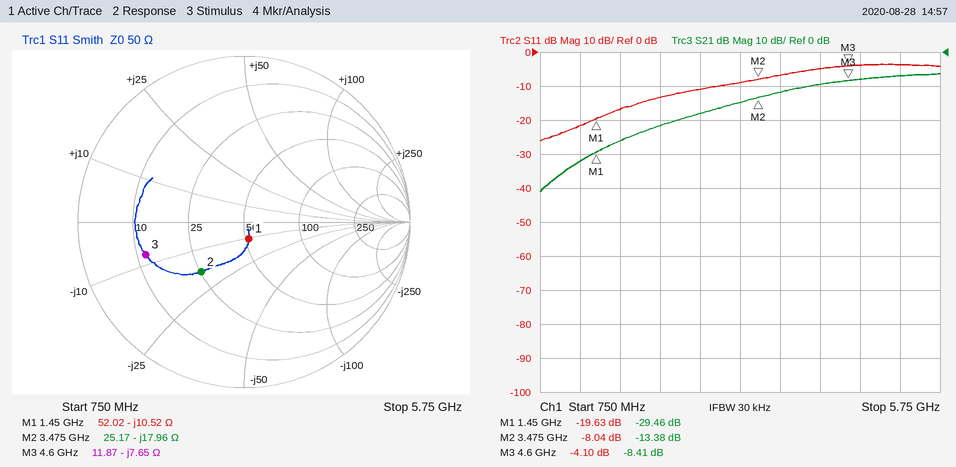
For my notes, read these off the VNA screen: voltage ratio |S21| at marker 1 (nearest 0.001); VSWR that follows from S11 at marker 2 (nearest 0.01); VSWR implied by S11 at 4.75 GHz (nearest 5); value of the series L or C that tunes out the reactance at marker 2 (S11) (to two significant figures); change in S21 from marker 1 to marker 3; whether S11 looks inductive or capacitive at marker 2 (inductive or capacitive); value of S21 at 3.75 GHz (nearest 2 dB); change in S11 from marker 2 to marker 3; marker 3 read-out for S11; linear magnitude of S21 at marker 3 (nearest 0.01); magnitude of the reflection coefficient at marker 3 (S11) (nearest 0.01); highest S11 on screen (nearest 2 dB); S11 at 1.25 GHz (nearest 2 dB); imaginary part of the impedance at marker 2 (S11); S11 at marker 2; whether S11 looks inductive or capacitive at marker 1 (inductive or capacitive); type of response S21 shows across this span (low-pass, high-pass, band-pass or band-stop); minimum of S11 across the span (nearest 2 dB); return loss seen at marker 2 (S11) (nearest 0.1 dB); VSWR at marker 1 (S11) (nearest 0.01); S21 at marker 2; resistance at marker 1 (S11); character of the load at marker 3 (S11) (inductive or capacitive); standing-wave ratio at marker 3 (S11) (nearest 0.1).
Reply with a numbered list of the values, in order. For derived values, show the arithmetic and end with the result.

1. 10^(-29.46/20) ≈ 0.034
2. (1 + 0.3963)/(1 − 0.3963) ≈ 2.31
3. |Γ| = 10^(-4/20) = 0.6310; VSWR = (1 + 0.6310)/(1 − 0.6310) ≈ 4.42, so 5 to the nearest 5
4. L = 17.96 Ω/(2π × 3.475 GHz) ≈ 823 pH, so 820 pH to two significant figures
5. -8.41 − (-29.46) = 21.05 dB
6. capacitive
7. -12 dB
8. -4.1 − (-8.04) = 3.94 dB
9. -4.10 dB
10. 10^(-8.41/20) ≈ 0.38
11. 10^(-4.1/20) ≈ 0.62
12. -4 dB
13. -22 dB
14. -17.96 Ω
15. -8.04 dB
16. capacitive
17. high-pass
18. -26 dB
19. 8.0 dB
20. (1 + 0.1044)/(1 − 0.1044) ≈ 1.23
21. -13.38 dB
22. 52.02 Ω
23. capacitive
24. 4.3
